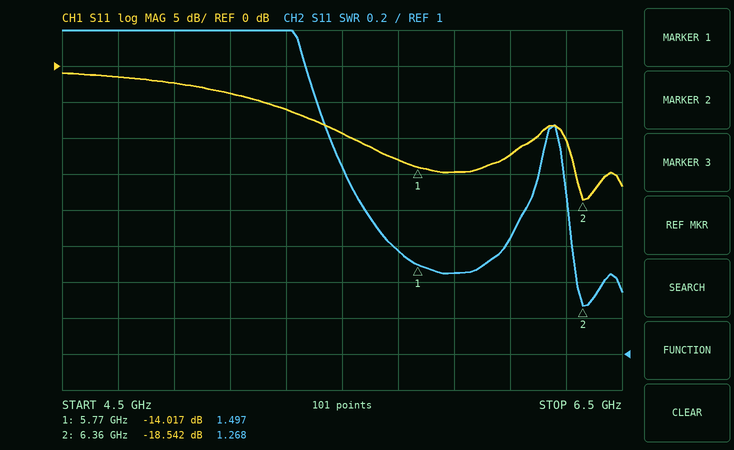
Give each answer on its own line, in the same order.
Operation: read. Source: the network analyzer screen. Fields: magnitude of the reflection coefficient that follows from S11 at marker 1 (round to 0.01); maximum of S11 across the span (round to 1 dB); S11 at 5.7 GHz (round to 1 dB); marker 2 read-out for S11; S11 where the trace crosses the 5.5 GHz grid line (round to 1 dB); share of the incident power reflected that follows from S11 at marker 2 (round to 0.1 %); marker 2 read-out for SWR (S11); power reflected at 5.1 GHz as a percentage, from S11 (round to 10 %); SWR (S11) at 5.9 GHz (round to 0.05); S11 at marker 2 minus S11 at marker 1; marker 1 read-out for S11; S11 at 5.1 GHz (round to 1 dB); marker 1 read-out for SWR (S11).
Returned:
0.20
-1 dB
-13 dB
-18.542 dB
-9 dB
1.4 %
1.268
40 %
1.45
-4.525 dB
-14.017 dB
-4 dB
1.497
